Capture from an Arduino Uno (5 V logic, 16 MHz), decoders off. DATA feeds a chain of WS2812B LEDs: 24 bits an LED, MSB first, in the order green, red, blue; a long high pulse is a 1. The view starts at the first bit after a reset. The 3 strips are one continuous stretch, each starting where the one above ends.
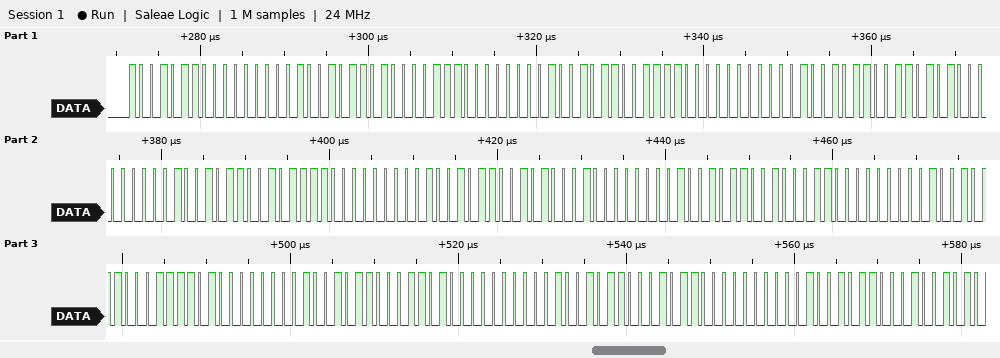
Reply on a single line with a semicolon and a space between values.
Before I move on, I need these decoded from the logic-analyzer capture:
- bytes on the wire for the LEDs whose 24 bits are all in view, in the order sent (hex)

96 00 96 87 00 96 78 00 96 6A 00 96 5E 00 96 51 00 96 46 00 96 3D 00 96 34 00 96 2C 00 96
